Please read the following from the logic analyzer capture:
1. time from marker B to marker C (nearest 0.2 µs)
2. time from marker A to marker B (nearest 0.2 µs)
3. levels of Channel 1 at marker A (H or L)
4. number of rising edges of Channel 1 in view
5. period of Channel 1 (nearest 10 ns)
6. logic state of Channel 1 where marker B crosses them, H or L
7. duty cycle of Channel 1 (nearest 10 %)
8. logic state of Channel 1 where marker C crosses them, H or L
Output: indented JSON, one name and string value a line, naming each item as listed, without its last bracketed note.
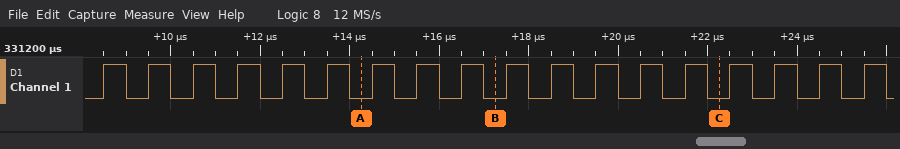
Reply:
{
  "time from marker B to marker C": "5 µs",
  "time from marker A to marker B": "3 µs",
  "levels of Channel 1 at marker A": "Channel 1=L",
  "number of rising edges of Channel 1 in view": "18",
  "period of Channel 1": "1000 ns",
  "logic state of Channel 1 where marker B crosses them, H or L": "Channel 1=L",
  "duty cycle of Channel 1": "50 %",
  "logic state of Channel 1 where marker C crosses them, H or L": "Channel 1=L"
}
